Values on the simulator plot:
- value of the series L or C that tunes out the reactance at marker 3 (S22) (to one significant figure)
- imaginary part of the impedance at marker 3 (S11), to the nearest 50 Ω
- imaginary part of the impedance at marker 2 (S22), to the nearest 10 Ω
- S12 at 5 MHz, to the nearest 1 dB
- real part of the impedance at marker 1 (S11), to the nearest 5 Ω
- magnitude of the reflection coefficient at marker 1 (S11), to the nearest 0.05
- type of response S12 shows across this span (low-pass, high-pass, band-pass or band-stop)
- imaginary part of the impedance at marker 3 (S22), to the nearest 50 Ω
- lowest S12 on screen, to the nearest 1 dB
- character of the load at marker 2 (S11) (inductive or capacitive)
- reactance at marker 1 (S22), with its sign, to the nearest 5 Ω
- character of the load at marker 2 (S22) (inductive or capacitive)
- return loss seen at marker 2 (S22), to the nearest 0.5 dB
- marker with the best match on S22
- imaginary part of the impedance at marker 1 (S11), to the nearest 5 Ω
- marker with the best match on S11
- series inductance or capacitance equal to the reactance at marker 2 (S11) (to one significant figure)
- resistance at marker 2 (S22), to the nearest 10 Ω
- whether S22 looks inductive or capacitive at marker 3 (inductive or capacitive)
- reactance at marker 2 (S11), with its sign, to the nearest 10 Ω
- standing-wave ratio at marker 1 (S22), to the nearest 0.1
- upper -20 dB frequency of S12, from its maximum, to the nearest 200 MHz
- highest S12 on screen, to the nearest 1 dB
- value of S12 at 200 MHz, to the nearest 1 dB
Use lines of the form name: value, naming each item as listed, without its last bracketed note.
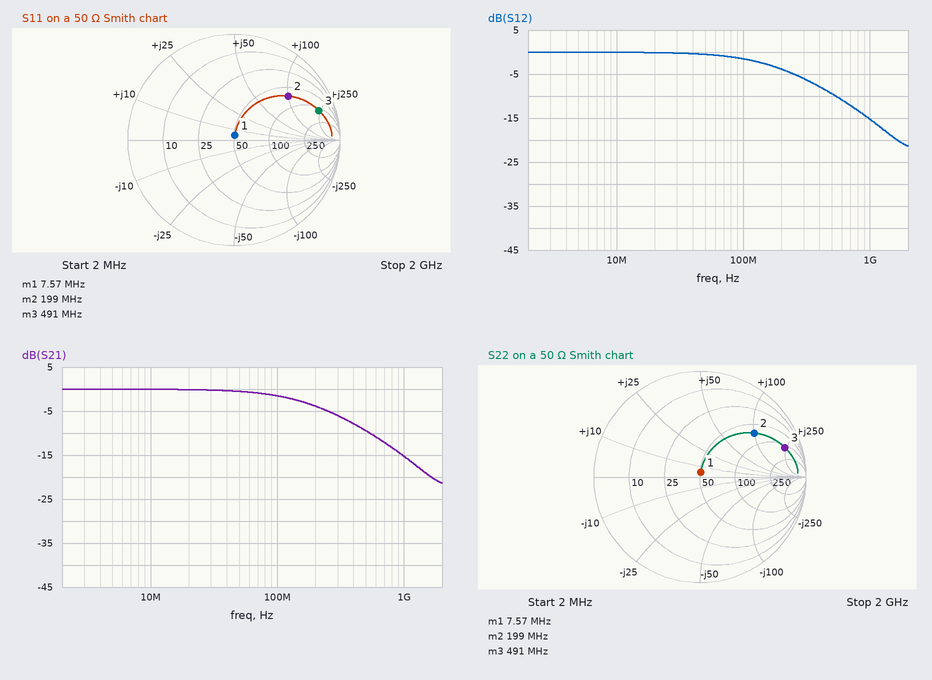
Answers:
value of the series L or C that tunes out the reactance at marker 3 (S22): 1 pF
imaginary part of the impedance at marker 3 (S11), to the nearest 50 Ω: +250 Ω
imaginary part of the impedance at marker 2 (S22), to the nearest 10 Ω: +100 Ω
S12 at 5 MHz, to the nearest 1 dB: 0 dB
real part of the impedance at marker 1 (S11), to the nearest 5 Ω: 50 Ω
magnitude of the reflection coefficient at marker 1 (S11), to the nearest 0.05: 0.05
type of response S12 shows across this span: low-pass
imaginary part of the impedance at marker 3 (S22), to the nearest 50 Ω: +250 Ω
lowest S12 on screen, to the nearest 1 dB: -21 dB
character of the load at marker 2 (S11): inductive
reactance at marker 1 (S22), with its sign, to the nearest 5 Ω: +5 Ω
character of the load at marker 2 (S22): inductive
return loss seen at marker 2 (S22), to the nearest 0.5 dB: 3.5 dB
marker with the best match on S22: marker 1
imaginary part of the impedance at marker 1 (S11), to the nearest 5 Ω: +5 Ω
marker with the best match on S11: marker 1
series inductance or capacitance equal to the reactance at marker 2 (S11): 80 nH
resistance at marker 2 (S22), to the nearest 10 Ω: 70 Ω
whether S22 looks inductive or capacitive at marker 3: inductive
reactance at marker 2 (S11), with its sign, to the nearest 10 Ω: +100 Ω
standing-wave ratio at marker 1 (S22), to the nearest 0.1: 1.1
upper -20 dB frequency of S12, from its maximum, to the nearest 200 MHz: 1.6 GHz
highest S12 on screen, to the nearest 1 dB: 0 dB
value of S12 at 200 MHz, to the nearest 1 dB: -4 dB
